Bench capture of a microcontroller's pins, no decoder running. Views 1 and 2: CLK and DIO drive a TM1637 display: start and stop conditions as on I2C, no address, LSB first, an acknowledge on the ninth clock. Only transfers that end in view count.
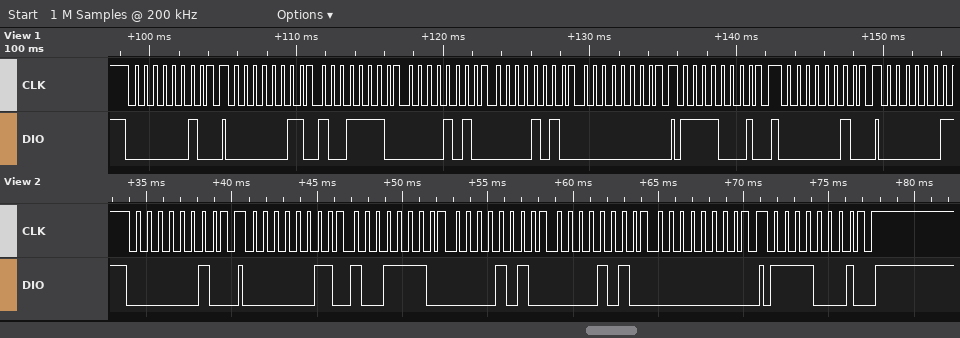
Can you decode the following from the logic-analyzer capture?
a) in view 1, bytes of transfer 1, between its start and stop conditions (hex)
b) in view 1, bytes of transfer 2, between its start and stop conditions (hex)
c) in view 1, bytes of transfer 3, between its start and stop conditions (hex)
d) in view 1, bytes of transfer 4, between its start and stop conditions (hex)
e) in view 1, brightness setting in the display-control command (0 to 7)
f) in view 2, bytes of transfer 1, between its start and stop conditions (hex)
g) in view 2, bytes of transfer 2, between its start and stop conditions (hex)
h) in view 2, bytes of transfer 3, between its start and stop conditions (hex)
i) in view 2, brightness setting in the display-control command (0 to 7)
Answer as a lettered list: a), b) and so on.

a) 40
b) C0 79 50 50 00
c) 8F
d) 40
e) 7
f) 40
g) C0 79 50 50 00
h) 8F
i) 7
